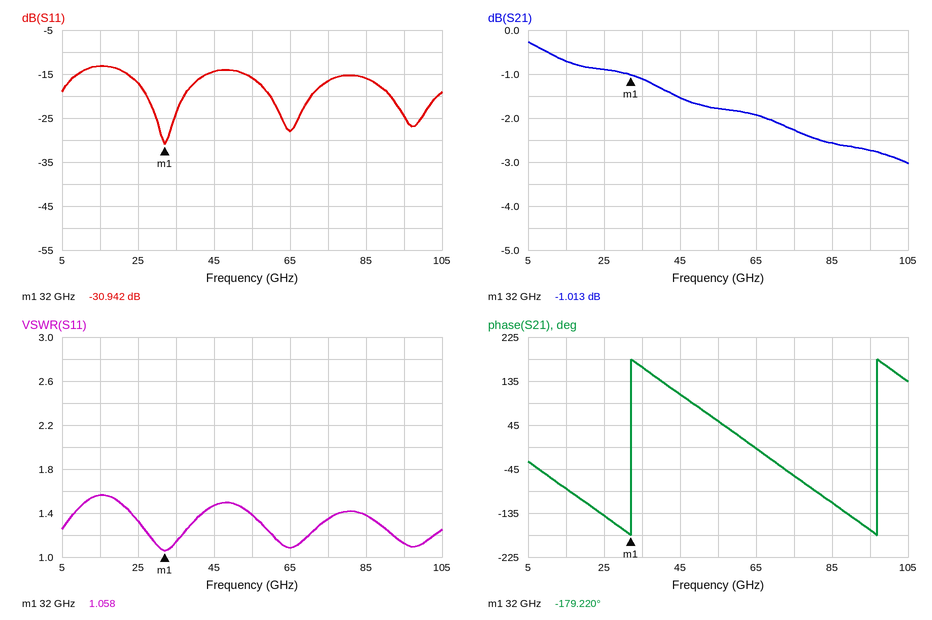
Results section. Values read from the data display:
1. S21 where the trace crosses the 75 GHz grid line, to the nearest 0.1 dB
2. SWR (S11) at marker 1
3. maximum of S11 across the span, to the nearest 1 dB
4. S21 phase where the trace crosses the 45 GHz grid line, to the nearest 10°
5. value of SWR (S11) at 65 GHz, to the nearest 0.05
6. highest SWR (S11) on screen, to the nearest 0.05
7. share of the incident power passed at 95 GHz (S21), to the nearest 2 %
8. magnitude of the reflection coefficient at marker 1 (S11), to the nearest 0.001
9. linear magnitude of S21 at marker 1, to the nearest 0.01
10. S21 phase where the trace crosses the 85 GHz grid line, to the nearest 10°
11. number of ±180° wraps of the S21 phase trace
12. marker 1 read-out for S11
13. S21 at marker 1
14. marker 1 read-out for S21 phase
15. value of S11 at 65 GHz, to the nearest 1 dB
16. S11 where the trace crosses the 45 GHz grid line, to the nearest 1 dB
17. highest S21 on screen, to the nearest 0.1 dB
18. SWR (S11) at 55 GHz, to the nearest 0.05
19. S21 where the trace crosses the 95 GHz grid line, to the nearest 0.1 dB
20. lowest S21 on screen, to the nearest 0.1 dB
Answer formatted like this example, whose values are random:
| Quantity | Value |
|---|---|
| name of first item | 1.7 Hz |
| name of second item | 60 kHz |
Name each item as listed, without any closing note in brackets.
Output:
| Quantity | Value |
|---|---|
| S21 where the trace crosses the 75 GHz grid line, to the nearest 0.1 dB | -2.3 dB |
| SWR (S11) at marker 1 | 1.058 |
| maximum of S11 across the span, to the nearest 1 dB | -13 dB |
| S21 phase where the trace crosses the 45 GHz grid line, to the nearest 10° | 110° |
| value of SWR (S11) at 65 GHz, to the nearest 0.05 | 1.10 |
| highest SWR (S11) on screen, to the nearest 0.05 | 1.55 |
| share of the incident power passed at 95 GHz (S21), to the nearest 2 % | 54 % |
| magnitude of the reflection coefficient at marker 1 (S11), to the nearest 0.001 | 0.028 |
| linear magnitude of S21 at marker 1, to the nearest 0.01 | 0.89 |
| S21 phase where the trace crosses the 85 GHz grid line, to the nearest 10° | -110° |
| number of ±180° wraps of the S21 phase trace | 2 |
| marker 1 read-out for S11 | -30.942 dB |
| S21 at marker 1 | -1.013 dB |
| marker 1 read-out for S21 phase | -179.220° |
| value of S11 at 65 GHz, to the nearest 1 dB | -28 dB |
| S11 where the trace crosses the 45 GHz grid line, to the nearest 1 dB | -14 dB |
| highest S21 on screen, to the nearest 0.1 dB | -0.3 dB |
| SWR (S11) at 55 GHz, to the nearest 0.05 | 1.40 |
| S21 where the trace crosses the 95 GHz grid line, to the nearest 0.1 dB | -2.7 dB |
| lowest S21 on screen, to the nearest 0.1 dB | -3.0 dB |
